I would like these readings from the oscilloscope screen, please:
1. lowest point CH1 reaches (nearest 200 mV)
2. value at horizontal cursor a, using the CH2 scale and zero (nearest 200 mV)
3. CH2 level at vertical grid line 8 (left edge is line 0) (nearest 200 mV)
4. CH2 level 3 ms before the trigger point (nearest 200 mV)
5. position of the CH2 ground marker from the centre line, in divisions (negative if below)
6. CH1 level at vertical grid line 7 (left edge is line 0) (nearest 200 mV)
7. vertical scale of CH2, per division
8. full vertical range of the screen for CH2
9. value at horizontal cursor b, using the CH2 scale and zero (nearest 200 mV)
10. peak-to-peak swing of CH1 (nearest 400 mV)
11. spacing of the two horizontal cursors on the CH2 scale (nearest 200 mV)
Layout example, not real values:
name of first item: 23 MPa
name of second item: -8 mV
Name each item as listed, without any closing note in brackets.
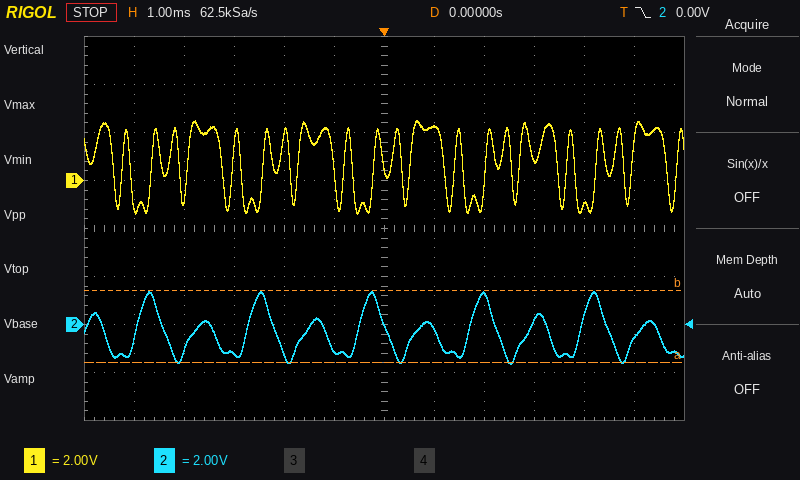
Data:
lowest point CH1 reaches: -1.4 V
value at horizontal cursor a, using the CH2 scale and zero: -1.6 V
CH2 level at vertical grid line 8 (left edge is line 0): 1.2 V
CH2 level 3 ms before the trigger point: -1.2 V
position of the CH2 ground marker from the centre line, in divisions: -2.0 div
CH1 level at vertical grid line 7 (left edge is line 0): 2.2 V
vertical scale of CH2, per division: 2 V
full vertical range of the screen for CH2: 16 V
value at horizontal cursor b, using the CH2 scale and zero: 1.4 V
peak-to-peak swing of CH1: 4.0 V
spacing of the two horizontal cursors on the CH2 scale: 3.0 V
